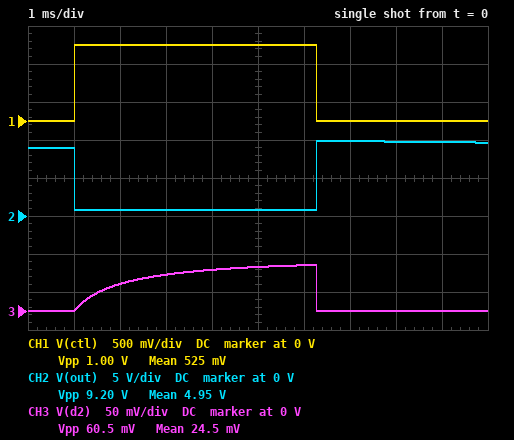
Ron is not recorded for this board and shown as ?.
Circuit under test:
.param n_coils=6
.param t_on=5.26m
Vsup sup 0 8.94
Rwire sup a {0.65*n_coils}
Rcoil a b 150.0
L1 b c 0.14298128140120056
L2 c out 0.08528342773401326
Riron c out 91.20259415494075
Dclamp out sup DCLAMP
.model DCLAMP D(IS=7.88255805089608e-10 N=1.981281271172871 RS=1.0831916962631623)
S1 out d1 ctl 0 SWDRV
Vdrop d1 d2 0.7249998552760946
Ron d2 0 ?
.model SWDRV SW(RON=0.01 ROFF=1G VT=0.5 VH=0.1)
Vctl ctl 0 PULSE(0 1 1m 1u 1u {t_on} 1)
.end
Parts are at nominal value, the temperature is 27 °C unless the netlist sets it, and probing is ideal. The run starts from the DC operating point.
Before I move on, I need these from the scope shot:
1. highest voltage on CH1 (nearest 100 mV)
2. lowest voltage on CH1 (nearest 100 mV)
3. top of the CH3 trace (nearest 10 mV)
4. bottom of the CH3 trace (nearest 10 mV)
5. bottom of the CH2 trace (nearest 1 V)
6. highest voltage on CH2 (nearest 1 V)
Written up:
1.0 V
0 V
60 mV
0 V
1 V
10 V
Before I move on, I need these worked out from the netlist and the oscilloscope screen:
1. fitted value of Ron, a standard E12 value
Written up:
1.2 Ω
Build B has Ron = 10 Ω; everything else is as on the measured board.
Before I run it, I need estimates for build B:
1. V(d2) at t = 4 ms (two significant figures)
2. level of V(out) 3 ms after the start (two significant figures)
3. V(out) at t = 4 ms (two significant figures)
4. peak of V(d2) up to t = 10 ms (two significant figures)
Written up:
430 mV
1.1 V
1.2 V
480 mV
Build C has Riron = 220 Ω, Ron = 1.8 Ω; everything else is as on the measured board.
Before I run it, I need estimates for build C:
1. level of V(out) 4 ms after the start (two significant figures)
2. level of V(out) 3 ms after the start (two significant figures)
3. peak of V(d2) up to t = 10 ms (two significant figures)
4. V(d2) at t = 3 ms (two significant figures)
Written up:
810 mV
800 mV
92 mV
70 mV
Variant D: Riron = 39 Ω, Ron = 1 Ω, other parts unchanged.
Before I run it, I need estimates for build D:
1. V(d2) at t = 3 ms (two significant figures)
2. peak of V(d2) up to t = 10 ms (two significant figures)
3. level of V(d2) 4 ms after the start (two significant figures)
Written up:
42 mV
50 mV
46 mV
